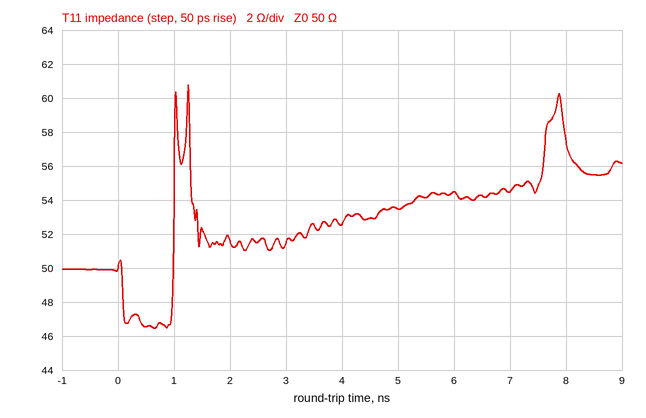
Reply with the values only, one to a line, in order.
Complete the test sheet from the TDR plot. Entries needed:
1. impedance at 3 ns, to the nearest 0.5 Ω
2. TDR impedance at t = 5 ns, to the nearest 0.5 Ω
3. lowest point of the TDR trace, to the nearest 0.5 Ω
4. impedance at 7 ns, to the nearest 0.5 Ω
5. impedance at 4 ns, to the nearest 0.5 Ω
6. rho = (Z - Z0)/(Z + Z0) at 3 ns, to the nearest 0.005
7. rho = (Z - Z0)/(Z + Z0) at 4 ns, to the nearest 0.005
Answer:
51.5 Ω
53.5 Ω
46.5 Ω
54.5 Ω
52.5 Ω
+0.015
+0.025
